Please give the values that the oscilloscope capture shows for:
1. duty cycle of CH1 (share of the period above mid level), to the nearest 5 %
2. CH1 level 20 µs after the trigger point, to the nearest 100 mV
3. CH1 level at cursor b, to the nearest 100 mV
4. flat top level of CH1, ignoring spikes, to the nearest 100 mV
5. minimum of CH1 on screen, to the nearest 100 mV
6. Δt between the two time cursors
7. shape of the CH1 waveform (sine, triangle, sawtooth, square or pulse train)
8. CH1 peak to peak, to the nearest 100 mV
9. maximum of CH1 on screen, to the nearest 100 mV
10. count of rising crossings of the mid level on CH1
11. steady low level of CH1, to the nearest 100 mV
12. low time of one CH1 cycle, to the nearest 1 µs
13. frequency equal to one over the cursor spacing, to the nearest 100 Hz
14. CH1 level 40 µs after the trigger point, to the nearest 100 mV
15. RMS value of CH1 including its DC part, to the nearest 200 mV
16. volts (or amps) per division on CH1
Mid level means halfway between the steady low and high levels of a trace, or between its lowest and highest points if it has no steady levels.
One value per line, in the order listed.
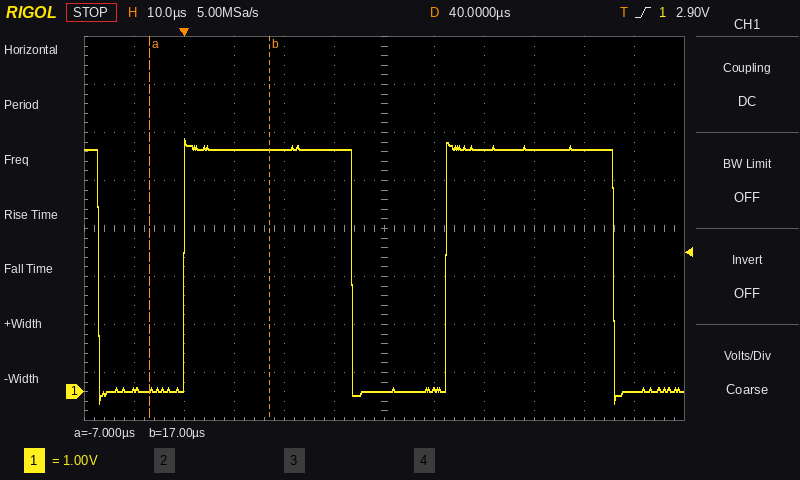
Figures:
65 %
5.0 V
5.0 V
5.0 V
-200 mV
24 µs
pulse train
5.5 V
5.3 V
2
0.0 V
18 µs
41.7 kHz
0.0 V
4.0 V
1 V
